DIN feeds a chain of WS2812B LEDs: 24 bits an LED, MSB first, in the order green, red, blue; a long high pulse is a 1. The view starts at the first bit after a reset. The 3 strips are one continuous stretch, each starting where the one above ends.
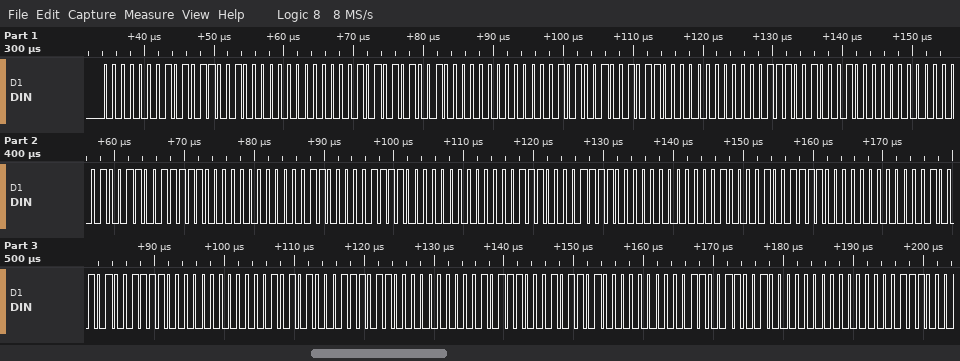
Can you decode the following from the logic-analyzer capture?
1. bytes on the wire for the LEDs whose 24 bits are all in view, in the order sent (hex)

01 59 00 05 52 00 0A 4B 00 0E 44 00 13 3E 00 18 3C 00 1C 3C 00 21 3C 00 25 3C 00 2A 3B 00 2E 2D 00 33 20 00
